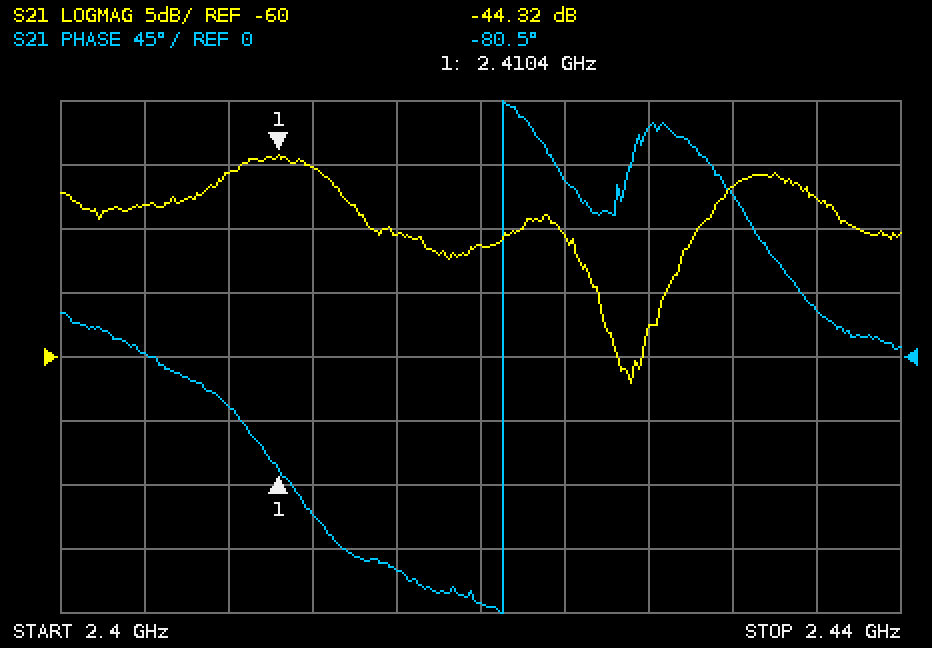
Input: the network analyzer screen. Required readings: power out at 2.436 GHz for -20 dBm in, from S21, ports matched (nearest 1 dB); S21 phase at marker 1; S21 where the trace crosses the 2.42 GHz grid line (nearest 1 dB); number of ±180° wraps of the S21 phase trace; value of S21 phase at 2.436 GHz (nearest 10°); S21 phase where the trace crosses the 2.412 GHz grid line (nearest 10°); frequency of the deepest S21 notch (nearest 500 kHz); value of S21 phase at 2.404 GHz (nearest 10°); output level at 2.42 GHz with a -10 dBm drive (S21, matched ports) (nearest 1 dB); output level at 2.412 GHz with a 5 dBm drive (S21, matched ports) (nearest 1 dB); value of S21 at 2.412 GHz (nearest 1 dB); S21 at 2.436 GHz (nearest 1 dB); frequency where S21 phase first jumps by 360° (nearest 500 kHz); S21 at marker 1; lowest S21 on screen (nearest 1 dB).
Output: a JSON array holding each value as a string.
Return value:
["-68 dBm", "-80.5°", "-51 dB", "1", "30°", "-110°", "2.4270 GHz", "0°", "-61 dBm", "-40 dBm", "-45 dB", "-48 dB", "2.4210 GHz", "-44.32 dB", "-62 dB"]
